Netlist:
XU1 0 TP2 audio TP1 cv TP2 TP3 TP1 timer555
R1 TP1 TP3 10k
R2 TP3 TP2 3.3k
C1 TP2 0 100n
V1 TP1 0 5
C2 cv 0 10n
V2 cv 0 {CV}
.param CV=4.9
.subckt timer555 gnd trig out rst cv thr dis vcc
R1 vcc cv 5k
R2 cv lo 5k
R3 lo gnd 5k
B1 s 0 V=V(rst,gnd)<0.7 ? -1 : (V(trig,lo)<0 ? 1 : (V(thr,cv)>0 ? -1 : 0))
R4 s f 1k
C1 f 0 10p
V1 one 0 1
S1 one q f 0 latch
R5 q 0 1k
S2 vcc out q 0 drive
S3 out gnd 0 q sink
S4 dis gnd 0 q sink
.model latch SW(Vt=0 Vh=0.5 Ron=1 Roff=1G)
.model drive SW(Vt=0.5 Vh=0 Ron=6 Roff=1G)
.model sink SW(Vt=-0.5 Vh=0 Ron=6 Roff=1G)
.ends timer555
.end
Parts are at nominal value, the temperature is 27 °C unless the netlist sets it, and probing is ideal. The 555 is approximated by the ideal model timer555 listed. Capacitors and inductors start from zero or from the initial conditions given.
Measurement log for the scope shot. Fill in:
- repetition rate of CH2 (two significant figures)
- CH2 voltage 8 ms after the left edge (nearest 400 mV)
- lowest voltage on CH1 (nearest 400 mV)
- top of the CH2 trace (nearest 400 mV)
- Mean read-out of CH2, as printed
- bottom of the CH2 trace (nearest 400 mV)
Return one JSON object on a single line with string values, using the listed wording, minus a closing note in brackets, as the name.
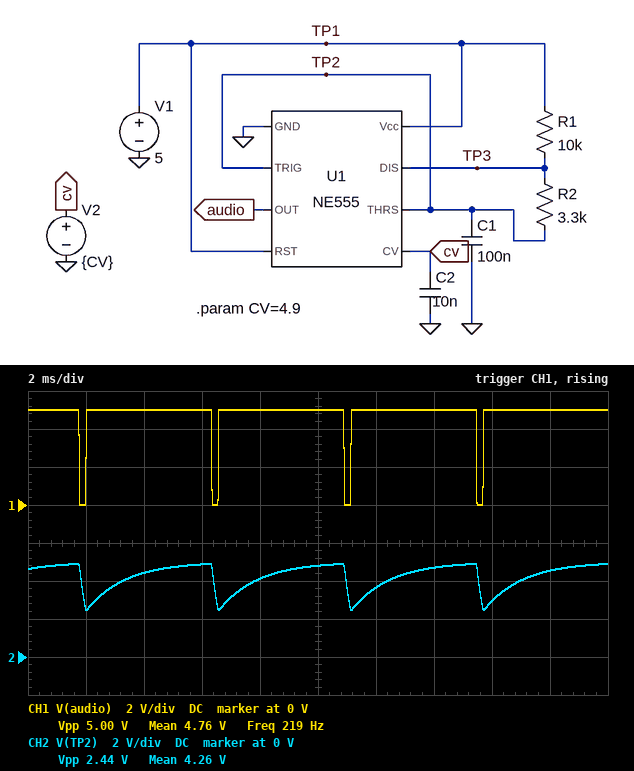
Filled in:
{"repetition rate of CH2": "220 Hz", "CH2 voltage 8 ms after the left edge": "4.0 V", "lowest voltage on CH1": "0 V", "top of the CH2 trace": "4.8 V", "Mean read-out of CH2, as printed": "4.26 V", "bottom of the CH2 trace": "2.4 V"}
